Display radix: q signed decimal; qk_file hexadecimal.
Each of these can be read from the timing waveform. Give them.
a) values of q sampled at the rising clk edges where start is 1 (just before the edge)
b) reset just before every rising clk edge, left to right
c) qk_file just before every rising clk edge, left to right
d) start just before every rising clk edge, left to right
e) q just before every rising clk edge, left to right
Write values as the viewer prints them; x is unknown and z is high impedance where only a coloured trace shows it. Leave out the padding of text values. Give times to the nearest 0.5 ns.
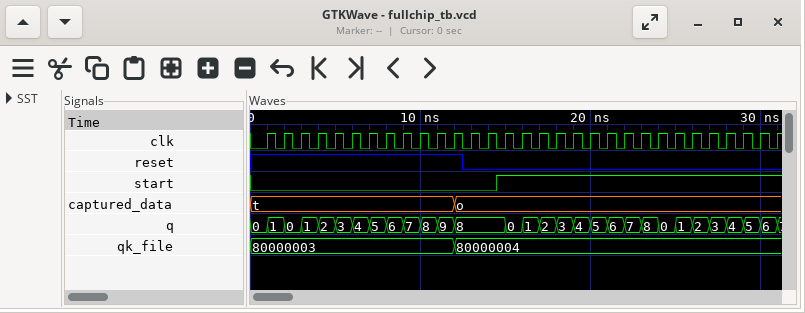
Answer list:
8, 0, 1, 2, 3, 4, 5, 6, 7, 8, 0, 1, 2, 3, 4, 5, 6
1 1 1 1 1 1 1 1 1 1 1 1 0 0 0 0 0 0 0 0 0 0 0 0 0 0 0 0 0 0 0
80000003, 80000003, 80000003, 80000003, 80000003, 80000003, 80000003, 80000003, 80000003, 80000003, 80000003, 80000003, 80000004, 80000004, 80000004, 80000004, 80000004, 80000004, 80000004, 80000004, 80000004, 80000004, 80000004, 80000004, 80000004, 80000004, 80000004, 80000004, 80000004, 80000004, 80000004
0 0 0 0 0 0 0 0 0 0 0 0 0 0 1 1 1 1 1 1 1 1 1 1 1 1 1 1 1 1 1
0, 1, 0, 1, 2, 3, 4, 5, 6, 7, 8, 9, 8, 8, 8, 0, 1, 2, 3, 4, 5, 6, 7, 8, 0, 1, 2, 3, 4, 5, 6
